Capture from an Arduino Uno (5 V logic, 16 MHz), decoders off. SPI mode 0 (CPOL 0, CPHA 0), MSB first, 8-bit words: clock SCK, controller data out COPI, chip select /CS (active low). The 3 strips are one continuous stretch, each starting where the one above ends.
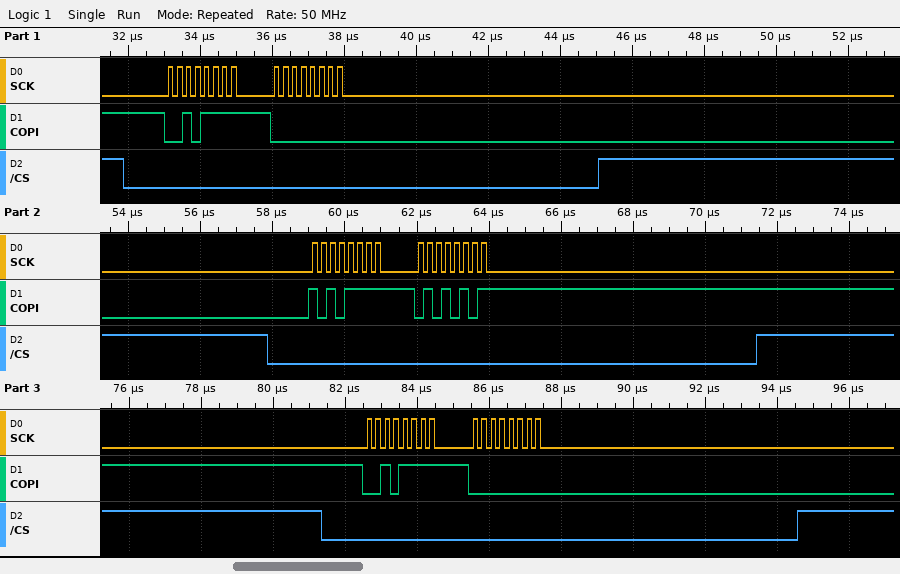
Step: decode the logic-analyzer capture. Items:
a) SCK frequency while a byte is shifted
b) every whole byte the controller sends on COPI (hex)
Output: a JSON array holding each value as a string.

["4 MHz", "0x2F 0x00 0xAF 0x55 0x2F 0x00"]
